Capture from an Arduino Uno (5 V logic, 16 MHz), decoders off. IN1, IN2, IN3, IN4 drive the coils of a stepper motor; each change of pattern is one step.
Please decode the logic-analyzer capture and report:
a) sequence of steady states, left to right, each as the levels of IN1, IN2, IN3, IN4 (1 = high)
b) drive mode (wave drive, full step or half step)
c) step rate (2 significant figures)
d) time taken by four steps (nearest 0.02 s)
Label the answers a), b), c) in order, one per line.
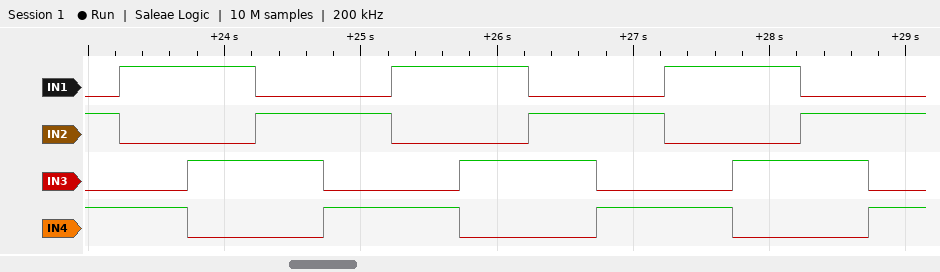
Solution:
a) 0101 1001 1010 0110 0101 1001 1010 0110 0101 1001 1010 0110 0101
b) full step
c) 2.0 steps/s
d) 2.00 s
